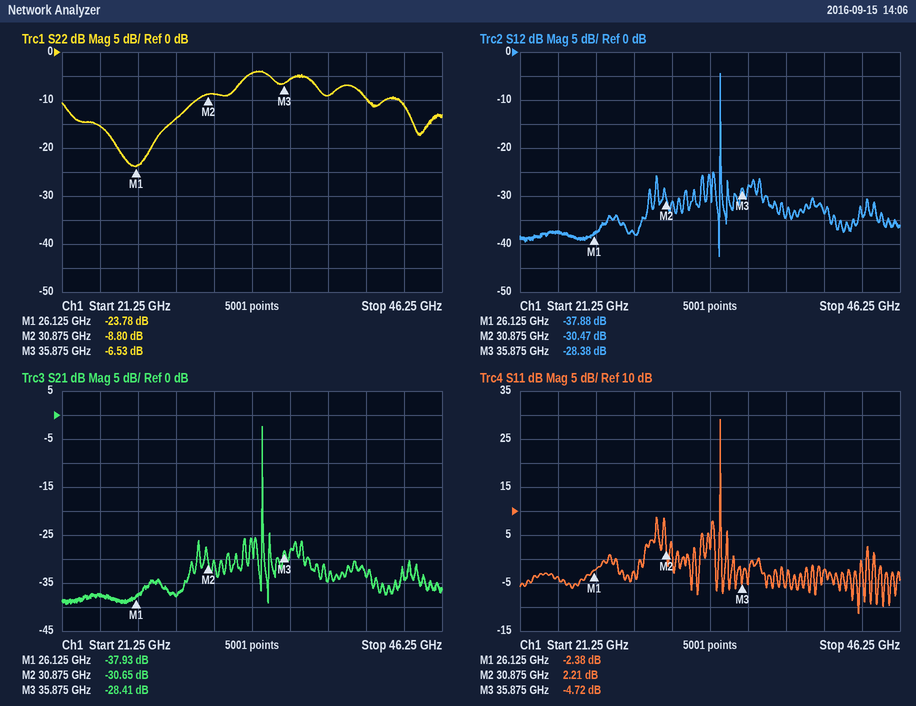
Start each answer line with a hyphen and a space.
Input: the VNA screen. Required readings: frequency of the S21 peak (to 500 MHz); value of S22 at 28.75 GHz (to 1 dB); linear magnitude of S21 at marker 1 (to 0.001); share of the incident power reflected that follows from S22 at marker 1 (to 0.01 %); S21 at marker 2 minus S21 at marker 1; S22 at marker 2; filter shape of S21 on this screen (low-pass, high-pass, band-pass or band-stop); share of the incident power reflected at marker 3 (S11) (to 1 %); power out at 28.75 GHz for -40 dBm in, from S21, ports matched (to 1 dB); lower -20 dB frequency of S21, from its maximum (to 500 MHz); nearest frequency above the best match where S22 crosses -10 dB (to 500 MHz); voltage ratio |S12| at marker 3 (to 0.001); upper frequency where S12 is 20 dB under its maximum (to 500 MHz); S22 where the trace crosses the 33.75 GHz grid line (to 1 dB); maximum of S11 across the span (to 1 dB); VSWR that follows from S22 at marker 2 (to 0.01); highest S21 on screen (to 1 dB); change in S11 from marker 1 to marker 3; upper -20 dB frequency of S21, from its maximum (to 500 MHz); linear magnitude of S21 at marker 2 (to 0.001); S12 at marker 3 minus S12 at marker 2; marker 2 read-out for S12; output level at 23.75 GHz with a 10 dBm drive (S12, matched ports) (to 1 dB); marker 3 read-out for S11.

- 34.5 GHz
- -14 dB
- 0.013
- 0.42 %
- 7.28 dB
- -8.80 dB
- band-pass
- 34 %
- -78 dBm
- 34.5 GHz
- 30.0 GHz
- 0.038
- 34.5 GHz
- -4 dB
- 29 dB
- 2.14
- -2 dB
- -2.34 dB
- 34.5 GHz
- 0.029
- 2.09 dB
- -30.47 dB
- -27 dBm
- -4.72 dB
